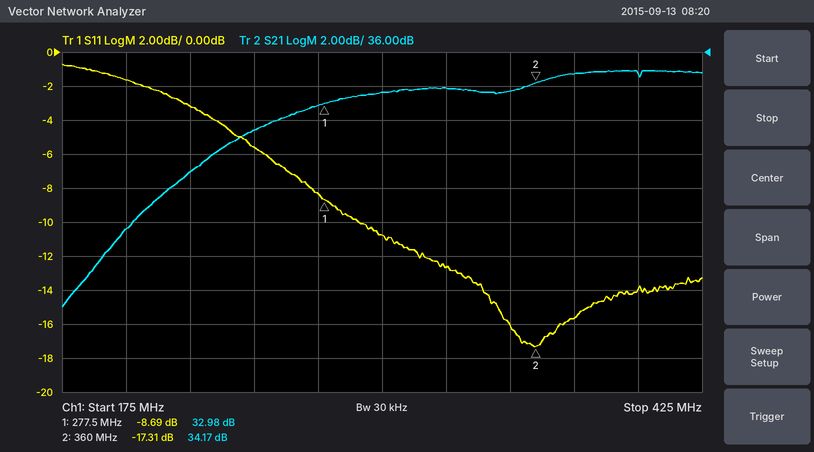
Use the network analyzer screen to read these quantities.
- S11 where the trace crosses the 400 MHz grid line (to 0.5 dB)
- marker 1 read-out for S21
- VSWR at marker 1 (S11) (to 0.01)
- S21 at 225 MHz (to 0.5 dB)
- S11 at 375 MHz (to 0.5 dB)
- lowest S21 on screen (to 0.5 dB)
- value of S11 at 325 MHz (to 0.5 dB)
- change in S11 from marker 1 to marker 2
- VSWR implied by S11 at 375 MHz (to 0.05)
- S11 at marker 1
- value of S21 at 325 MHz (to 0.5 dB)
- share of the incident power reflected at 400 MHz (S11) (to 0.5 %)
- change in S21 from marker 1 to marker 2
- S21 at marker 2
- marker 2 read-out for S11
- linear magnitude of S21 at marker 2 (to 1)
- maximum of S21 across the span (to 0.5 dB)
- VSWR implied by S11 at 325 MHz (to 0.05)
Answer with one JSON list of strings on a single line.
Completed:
["-14.0 dB", "32.98 dB", "2.16", "29.0 dB", "-15.5 dB", "21.0 dB", "-12.5 dB", "-8.62 dB", "1.40", "-8.69 dB", "34.0 dB", "4.0 %", "1.19 dB", "34.17 dB", "-17.31 dB", "51", "35.0 dB", "1.60"]
